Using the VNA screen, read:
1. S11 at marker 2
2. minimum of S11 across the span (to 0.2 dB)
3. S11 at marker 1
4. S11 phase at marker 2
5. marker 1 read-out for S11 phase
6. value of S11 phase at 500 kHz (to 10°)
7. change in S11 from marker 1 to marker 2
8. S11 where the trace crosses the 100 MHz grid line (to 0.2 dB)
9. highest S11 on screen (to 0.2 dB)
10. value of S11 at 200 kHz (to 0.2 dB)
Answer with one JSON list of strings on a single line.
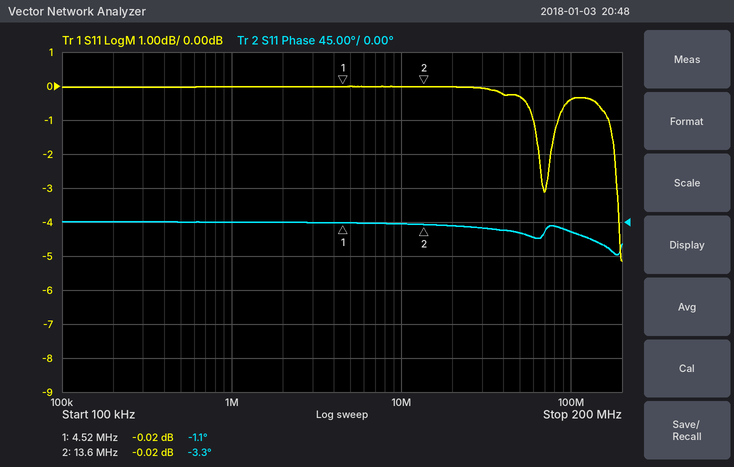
["-0.02 dB", "-5.2 dB", "-0.02 dB", "-3.3°", "-1.1°", "0°", "0.00 dB", "-0.4 dB", "0.0 dB", "0.0 dB"]
